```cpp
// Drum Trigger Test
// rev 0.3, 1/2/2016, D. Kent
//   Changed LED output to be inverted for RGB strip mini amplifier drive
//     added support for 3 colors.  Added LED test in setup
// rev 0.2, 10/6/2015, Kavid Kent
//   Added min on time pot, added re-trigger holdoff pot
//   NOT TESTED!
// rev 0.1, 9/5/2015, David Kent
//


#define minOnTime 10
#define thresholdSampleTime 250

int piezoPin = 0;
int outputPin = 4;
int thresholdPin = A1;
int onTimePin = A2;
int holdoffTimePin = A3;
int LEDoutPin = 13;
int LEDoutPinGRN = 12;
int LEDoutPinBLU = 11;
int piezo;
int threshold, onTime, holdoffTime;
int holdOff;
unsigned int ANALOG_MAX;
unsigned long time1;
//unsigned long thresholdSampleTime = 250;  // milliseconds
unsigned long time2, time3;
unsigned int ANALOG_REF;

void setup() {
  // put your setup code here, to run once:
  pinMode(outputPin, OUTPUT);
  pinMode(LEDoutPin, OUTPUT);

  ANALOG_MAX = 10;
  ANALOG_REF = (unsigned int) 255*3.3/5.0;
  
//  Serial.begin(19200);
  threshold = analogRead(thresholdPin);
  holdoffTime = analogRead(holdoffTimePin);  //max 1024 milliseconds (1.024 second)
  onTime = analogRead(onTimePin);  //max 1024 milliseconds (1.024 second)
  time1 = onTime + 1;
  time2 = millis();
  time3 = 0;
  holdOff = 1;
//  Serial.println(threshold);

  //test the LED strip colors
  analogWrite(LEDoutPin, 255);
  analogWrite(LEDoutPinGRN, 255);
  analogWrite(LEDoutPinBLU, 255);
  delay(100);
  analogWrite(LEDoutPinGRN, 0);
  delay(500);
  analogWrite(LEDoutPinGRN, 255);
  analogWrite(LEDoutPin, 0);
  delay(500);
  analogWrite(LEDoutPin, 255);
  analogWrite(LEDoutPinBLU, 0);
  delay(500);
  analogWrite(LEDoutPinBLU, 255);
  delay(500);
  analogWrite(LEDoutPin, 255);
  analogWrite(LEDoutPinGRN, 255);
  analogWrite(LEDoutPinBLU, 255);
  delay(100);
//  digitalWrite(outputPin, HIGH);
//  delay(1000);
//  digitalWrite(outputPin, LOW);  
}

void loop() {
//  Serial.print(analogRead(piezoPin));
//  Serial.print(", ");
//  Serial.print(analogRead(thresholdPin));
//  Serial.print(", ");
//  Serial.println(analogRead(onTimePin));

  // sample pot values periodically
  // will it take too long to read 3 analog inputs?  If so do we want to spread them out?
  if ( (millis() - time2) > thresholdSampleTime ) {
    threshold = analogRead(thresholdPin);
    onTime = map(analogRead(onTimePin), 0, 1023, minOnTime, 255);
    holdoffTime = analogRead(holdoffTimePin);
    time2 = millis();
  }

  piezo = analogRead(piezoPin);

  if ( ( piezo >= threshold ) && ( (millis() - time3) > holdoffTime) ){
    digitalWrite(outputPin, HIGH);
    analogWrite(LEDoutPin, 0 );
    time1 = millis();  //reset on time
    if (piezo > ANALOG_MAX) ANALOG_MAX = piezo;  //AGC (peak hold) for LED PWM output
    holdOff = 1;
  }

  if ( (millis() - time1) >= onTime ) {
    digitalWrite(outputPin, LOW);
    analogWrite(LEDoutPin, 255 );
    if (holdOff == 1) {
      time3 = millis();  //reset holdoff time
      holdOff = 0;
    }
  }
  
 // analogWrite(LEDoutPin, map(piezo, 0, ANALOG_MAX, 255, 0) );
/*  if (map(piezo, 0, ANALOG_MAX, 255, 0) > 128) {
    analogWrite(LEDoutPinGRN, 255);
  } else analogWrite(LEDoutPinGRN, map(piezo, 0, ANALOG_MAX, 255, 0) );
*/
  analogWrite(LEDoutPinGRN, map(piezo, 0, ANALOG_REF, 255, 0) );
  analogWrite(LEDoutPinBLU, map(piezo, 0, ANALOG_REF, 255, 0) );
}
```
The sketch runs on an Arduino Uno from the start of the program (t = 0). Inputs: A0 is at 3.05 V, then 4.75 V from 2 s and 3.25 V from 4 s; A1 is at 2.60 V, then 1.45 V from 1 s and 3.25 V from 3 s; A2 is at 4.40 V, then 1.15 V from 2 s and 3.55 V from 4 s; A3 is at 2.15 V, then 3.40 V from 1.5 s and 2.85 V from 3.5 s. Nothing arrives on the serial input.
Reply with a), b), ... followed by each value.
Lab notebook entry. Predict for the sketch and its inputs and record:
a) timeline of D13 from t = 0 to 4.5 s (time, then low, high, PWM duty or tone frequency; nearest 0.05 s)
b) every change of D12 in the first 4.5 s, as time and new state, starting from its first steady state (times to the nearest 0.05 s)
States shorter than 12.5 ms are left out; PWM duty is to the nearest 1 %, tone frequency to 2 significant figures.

a) 0 s high; 0.6 s low; 1.1 s high; 2.2 s low
b) 0 s high; 0.1 s low; 0.6 s high; 2.2 s low
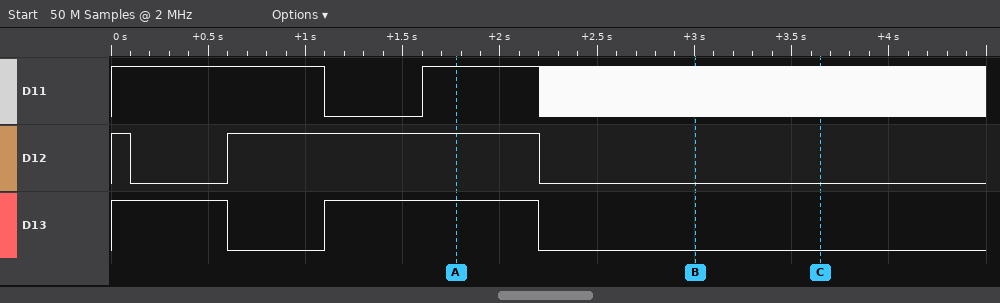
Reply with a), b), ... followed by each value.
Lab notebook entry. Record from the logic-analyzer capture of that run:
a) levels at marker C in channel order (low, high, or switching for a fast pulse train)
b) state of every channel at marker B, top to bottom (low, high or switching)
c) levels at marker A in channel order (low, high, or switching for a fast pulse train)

a) D11 switching, D12 low, D13 low
b) D11 switching, D12 low, D13 low
c) D11 high, D12 high, D13 high
